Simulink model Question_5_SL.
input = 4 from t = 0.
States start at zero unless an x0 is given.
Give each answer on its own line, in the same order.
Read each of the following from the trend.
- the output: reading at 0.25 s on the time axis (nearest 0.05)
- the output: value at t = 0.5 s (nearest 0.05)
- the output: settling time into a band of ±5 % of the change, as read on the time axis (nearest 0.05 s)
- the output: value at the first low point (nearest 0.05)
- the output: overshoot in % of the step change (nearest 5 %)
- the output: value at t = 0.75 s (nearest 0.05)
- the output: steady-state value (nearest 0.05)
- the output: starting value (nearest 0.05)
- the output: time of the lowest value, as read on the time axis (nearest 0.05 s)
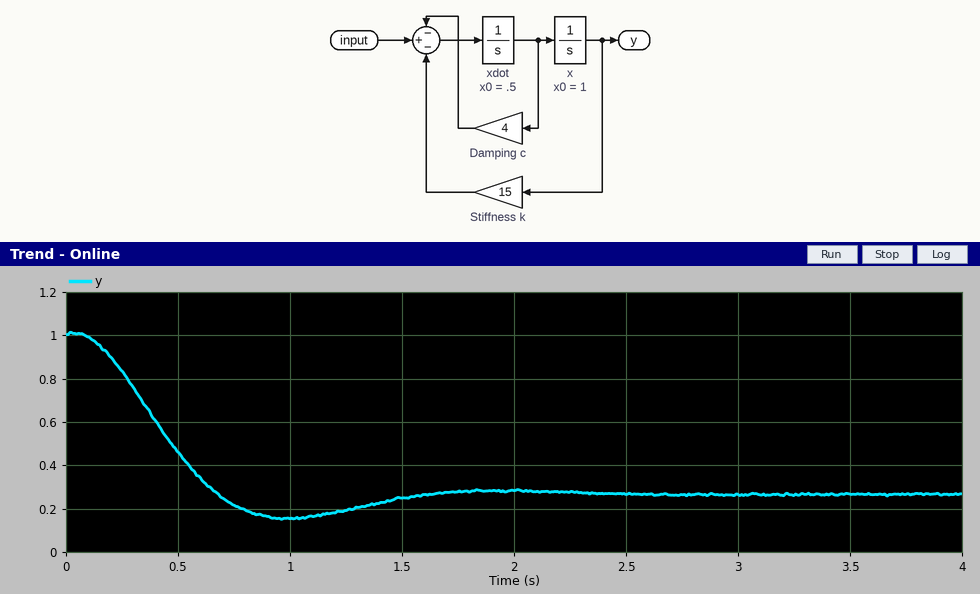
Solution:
0.85
0.45
1.40 s
0.15
15 %
0.20
0.25
1.00
1.00 s
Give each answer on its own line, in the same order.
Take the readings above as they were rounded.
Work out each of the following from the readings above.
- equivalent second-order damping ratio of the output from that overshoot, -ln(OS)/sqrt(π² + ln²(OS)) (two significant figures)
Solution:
0.52
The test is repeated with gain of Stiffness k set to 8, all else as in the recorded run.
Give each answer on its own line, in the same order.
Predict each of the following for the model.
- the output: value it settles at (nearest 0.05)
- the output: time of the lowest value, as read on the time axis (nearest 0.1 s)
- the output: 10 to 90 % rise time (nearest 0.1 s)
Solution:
0.50
1.7 s
0.7 s
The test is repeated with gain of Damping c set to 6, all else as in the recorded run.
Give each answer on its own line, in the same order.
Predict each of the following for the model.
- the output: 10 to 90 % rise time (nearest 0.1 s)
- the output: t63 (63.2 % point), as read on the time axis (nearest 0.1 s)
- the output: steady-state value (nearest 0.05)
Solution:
0.6 s
0.5 s
0.25
